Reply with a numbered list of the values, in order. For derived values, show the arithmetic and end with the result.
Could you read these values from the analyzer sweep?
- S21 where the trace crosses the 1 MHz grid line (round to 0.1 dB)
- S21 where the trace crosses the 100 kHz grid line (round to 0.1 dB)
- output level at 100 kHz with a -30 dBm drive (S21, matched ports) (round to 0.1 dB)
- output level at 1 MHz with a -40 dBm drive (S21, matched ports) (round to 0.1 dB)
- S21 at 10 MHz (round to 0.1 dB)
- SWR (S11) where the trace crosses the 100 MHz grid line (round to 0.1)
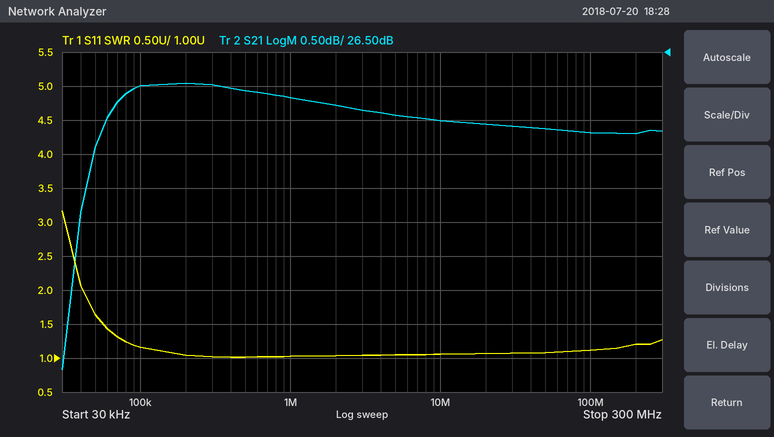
1. 25.8 dB
2. 26.0 dB
3. -30 dBm + (26.0 dB) = -4.0 dBm
4. -40 dBm + (25.8 dB) = -14.2 dBm
5. 25.5 dB
6. 1.1
